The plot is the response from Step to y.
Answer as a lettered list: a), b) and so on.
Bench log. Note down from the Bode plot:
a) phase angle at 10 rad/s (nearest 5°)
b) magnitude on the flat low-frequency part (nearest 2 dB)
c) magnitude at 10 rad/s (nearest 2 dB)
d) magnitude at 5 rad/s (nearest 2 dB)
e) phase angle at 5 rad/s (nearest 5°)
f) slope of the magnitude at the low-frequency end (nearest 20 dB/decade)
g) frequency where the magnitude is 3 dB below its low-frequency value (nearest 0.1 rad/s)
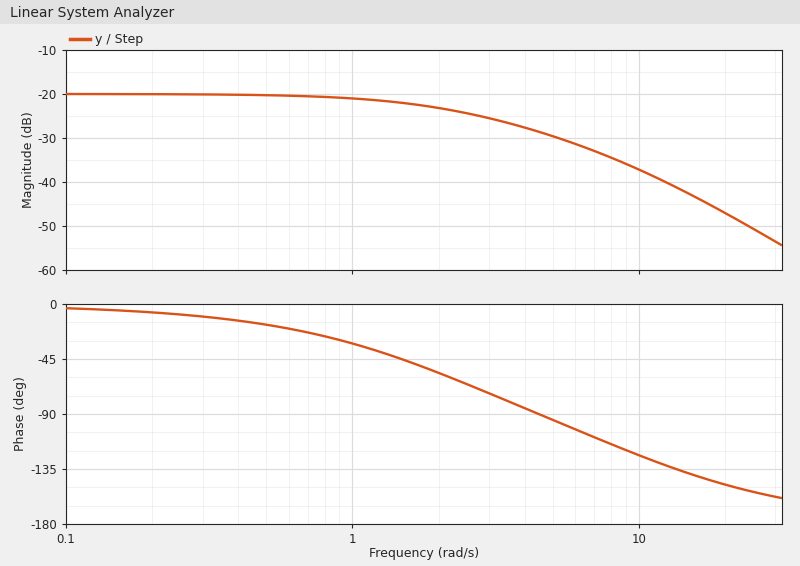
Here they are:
a) -125°
b) -20 dB
c) -38 dB
d) -30 dB
e) -95°
f) 0 dB/decade
g) 1.9 rad/s
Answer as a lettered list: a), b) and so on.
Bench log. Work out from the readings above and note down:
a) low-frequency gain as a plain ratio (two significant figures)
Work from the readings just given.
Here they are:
a) 0.10
